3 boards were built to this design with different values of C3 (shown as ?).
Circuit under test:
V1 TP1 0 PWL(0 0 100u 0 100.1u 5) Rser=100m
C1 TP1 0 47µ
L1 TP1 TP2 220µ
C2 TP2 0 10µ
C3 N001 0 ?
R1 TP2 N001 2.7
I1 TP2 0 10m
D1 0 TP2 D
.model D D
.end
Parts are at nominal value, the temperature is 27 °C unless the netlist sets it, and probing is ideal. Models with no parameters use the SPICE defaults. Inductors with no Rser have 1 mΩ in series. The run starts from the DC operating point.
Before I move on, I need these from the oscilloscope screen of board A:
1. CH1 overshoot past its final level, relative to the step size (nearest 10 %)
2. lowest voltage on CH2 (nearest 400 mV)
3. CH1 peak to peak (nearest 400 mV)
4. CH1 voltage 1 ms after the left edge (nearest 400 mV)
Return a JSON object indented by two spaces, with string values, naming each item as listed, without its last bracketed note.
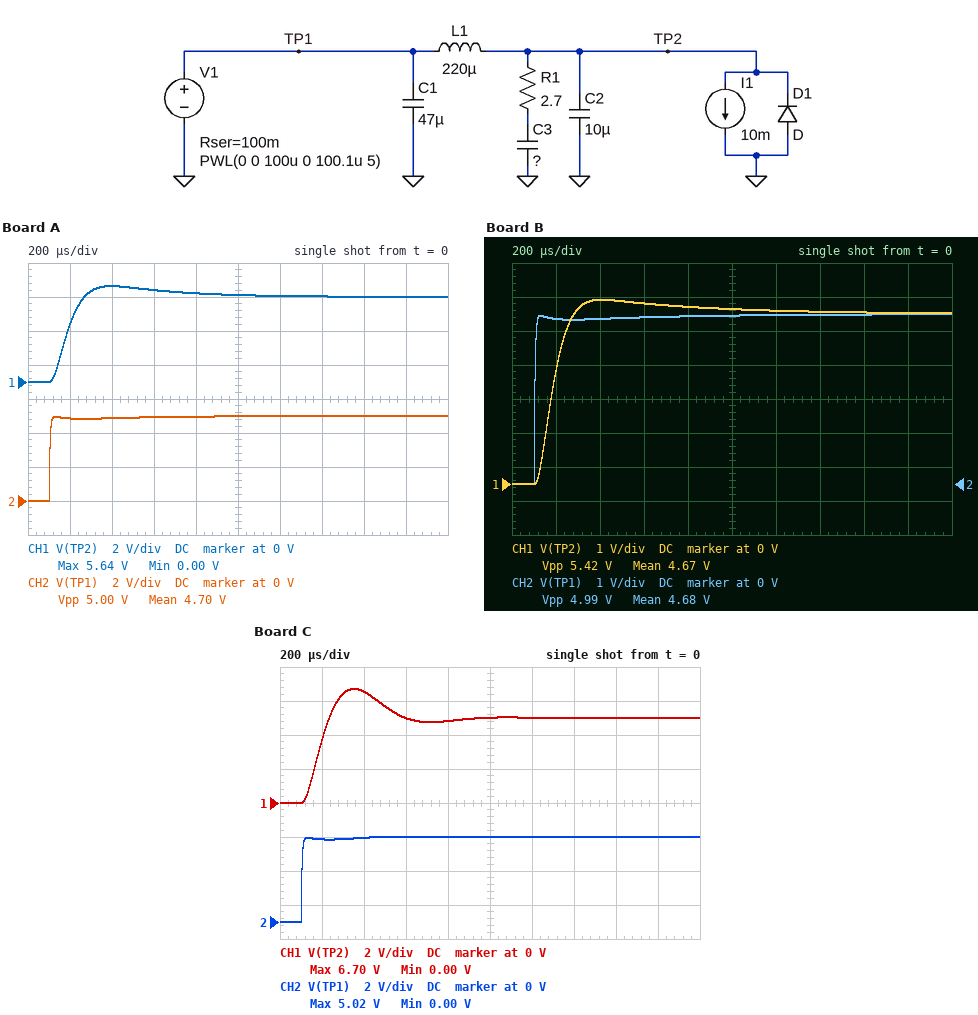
{
  "CH1 overshoot past its final level, relative to the step size": "10 %",
  "lowest voltage on CH2": "0 V",
  "CH1 peak to peak": "5.6 V",
  "CH1 voltage 1 ms after the left edge": "5.2 V"
}
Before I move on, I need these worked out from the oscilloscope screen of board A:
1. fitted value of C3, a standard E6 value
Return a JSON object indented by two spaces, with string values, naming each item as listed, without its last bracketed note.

{
  "fitted value of C3, a standard E6 value": "150 µF"
}
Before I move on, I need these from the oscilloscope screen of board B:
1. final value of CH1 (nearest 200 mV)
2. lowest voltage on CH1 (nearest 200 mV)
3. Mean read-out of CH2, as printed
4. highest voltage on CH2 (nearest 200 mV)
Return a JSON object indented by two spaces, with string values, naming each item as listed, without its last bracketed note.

{
  "final value of CH1": "5.0 V",
  "lowest voltage on CH1": "0 V",
  "Mean read-out of CH2, as printed": "4.68 V",
  "highest voltage on CH2": "5.0 V"
}
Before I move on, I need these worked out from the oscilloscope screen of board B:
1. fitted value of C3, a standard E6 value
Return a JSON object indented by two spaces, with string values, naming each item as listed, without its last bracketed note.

{
  "fitted value of C3, a standard E6 value": "220 µF"
}
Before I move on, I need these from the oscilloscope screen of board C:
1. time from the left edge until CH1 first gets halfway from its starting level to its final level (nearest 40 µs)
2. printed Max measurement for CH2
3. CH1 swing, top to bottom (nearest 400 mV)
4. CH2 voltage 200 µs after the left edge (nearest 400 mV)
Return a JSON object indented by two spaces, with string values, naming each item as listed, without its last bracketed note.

{
  "time from the left edge until CH1 first gets halfway from its starting level to its final level": "160 µs",
  "printed Max measurement for CH2": "5.02 V",
  "CH1 swing, top to bottom": "6.8 V",
  "CH2 voltage 200 µs after the left edge": "4.8 V"
}
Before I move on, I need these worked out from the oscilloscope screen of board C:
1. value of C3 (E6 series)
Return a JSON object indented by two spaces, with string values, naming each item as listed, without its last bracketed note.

{
  "value of C3": "47 µF"
}
